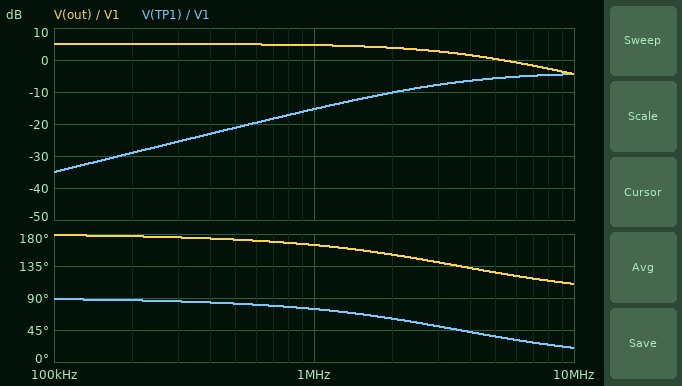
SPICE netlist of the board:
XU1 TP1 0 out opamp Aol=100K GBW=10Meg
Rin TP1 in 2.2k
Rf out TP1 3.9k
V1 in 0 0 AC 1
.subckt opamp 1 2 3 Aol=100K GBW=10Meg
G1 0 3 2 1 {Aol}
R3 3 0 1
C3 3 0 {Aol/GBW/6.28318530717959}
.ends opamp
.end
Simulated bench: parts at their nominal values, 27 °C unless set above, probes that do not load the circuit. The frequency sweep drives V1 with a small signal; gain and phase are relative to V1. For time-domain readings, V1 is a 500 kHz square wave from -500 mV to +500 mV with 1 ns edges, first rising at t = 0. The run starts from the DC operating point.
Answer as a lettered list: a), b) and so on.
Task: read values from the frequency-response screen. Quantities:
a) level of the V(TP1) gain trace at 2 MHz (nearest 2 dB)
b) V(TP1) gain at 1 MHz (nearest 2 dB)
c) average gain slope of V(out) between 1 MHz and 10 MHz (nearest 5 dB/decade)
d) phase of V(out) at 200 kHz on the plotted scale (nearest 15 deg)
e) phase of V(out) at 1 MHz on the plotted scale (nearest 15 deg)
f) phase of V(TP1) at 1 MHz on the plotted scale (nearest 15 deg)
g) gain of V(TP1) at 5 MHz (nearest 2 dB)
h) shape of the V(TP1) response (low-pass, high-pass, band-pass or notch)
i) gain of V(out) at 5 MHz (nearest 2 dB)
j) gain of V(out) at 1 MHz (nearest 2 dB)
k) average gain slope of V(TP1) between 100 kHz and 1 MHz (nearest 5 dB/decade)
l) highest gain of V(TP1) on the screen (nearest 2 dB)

a) -10 dB
b) -16 dB
c) -10 dB/decade
d) 180 deg
e) 165 deg
f) 75 deg
g) -6 dB
h) high-pass
i) 0 dB
j) 4 dB
k) 20 dB/decade
l) -4 dB
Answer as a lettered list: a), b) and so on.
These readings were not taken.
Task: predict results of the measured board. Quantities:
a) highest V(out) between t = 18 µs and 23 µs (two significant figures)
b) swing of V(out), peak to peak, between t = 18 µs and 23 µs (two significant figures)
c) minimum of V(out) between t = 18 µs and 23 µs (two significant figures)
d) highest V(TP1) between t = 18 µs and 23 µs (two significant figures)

a) 890 mV
b) 1.8 V
c) -890 mV
d) 630 mV
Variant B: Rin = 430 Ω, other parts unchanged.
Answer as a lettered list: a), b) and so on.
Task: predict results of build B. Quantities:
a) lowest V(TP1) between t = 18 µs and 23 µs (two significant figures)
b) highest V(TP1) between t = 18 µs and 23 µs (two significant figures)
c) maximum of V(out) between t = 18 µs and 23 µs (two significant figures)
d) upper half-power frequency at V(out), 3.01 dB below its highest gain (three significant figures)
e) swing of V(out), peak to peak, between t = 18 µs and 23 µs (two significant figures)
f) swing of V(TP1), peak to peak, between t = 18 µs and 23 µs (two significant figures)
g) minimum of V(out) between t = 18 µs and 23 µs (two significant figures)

a) -900 mV
b) 900 mV
c) 4.5 V
d) 993 kHz
e) 9.0 V
f) 1.8 V
g) -4.5 V
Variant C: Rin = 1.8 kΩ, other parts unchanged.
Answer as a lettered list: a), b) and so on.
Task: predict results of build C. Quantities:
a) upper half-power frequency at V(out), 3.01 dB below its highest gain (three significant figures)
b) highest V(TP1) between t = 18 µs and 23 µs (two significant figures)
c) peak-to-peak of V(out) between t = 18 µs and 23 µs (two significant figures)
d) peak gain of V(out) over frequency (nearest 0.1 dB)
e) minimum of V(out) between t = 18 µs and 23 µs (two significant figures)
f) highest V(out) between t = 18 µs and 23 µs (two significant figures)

a) 3.16 MHz
b) 680 mV
c) 2.2 V
d) 6.7 dB
e) -1.1 V
f) 1.1 V
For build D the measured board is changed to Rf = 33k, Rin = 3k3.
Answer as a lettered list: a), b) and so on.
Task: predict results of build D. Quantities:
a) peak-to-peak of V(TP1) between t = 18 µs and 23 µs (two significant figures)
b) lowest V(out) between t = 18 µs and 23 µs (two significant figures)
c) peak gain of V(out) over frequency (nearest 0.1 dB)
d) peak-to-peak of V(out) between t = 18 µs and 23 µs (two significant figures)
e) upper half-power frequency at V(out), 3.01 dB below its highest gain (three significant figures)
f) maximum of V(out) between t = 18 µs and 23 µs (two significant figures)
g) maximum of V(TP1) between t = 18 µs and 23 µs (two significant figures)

a) 1.8 V
b) -5.0 V
c) 20.0 dB
d) 9.9 V
e) 909 kHz
f) 5.0 V
g) 900 mV
